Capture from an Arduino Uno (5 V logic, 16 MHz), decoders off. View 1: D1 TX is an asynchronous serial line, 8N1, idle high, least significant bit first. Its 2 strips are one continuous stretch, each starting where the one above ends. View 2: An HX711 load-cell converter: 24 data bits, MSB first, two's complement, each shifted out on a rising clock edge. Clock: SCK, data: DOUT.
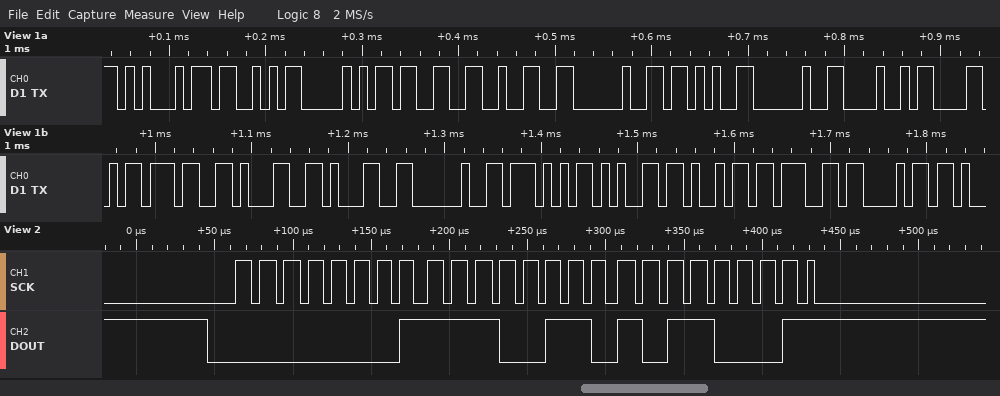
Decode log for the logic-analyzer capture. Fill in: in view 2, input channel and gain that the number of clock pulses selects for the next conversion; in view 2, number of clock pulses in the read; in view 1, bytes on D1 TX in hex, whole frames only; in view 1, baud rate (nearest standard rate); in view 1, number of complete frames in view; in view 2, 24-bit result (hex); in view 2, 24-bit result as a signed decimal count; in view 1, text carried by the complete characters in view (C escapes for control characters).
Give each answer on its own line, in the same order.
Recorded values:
channel A, gain 128
25
0x45 0x53 0x50 0x33 0x32 0x20 0x2B 0x20 0x48 0x58 0x37 0x31 0x31 0x20 0x57 0x65 0x69 0x67 0x68
115200 baud
19
0x01E6B1
124593
"ESP32 + HX711 Weigh"
